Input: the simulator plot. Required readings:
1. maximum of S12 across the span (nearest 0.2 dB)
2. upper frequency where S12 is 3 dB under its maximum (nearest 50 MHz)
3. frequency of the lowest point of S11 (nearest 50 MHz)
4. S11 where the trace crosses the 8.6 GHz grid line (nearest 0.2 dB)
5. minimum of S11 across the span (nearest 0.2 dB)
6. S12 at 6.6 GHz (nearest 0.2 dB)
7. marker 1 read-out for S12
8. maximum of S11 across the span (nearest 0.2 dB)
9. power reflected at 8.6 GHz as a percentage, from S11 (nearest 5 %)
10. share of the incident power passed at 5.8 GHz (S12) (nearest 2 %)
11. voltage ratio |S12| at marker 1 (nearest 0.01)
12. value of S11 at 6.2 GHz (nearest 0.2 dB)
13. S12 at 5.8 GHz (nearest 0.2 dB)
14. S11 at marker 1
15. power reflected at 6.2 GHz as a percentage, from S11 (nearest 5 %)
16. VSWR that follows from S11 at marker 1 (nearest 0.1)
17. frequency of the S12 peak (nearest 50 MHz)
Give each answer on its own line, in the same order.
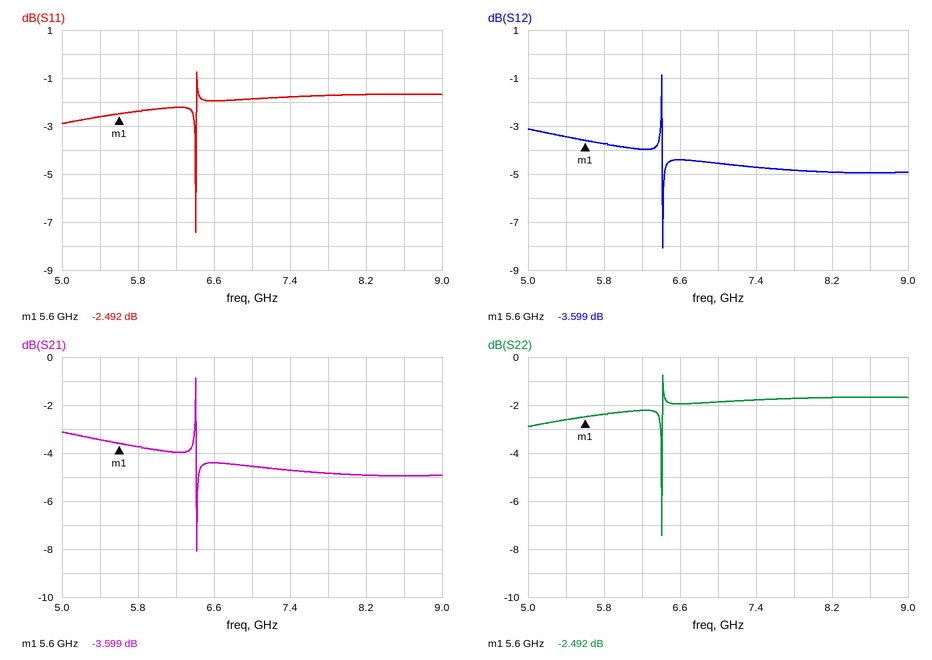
-0.8 dB
6.40 GHz
6.40 GHz
-1.6 dB
-7.4 dB
-4.4 dB
-3.599 dB
-0.8 dB
70 %
42 %
0.66
-2.2 dB
-3.8 dB
-2.492 dB
60 %
7.0
6.40 GHz
